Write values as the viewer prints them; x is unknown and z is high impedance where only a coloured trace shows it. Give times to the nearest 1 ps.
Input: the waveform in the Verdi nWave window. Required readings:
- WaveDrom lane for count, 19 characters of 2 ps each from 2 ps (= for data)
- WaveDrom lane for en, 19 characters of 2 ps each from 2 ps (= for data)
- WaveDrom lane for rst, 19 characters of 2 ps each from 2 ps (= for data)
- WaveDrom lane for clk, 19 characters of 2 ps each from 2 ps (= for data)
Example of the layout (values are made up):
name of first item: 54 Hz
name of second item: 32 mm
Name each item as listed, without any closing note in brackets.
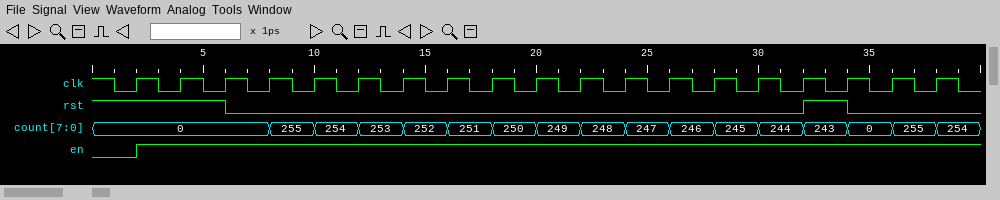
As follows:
WaveDrom lane for count, 19 characters of 2 ps each from 2 ps: {name: 'count', wave: '=..================', data: '0 255 254 253 252 251 250 249 248 247 246 245 244 243 0 255 254'}
WaveDrom lane for en, 19 characters of 2 ps each from 2 ps: {name: 'en', wave: '1..................'}
WaveDrom lane for rst, 19 characters of 2 ps each from 2 ps: {name: 'rst', wave: '1.0............10..'}
WaveDrom lane for clk, 19 characters of 2 ps each from 2 ps: {name: 'clk', wave: 'p..................'}
